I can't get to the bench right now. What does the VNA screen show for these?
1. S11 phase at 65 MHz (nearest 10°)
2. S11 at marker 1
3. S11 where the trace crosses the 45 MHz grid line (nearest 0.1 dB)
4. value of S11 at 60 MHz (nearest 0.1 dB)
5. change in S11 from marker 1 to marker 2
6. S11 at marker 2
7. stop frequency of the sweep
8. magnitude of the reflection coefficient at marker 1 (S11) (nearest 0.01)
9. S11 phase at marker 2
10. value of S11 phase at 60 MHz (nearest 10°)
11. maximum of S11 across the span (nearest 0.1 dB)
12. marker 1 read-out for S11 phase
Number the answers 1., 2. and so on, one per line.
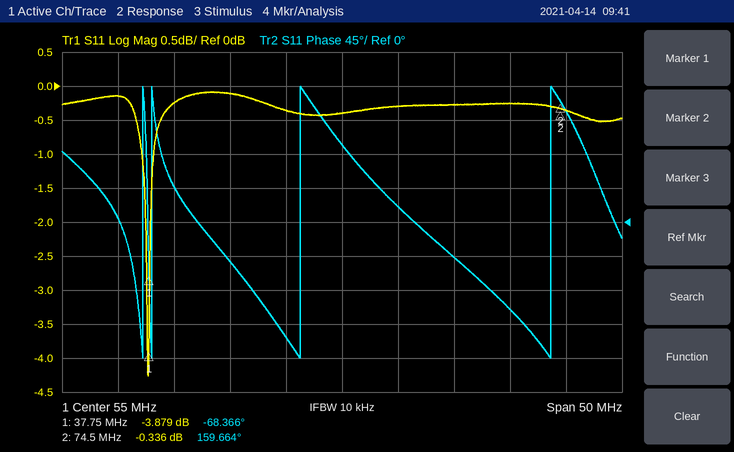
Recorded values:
1. -50°
2. -3.879 dB
3. -0.1 dB
4. -0.3 dB
5. 3.543 dB
6. -0.336 dB
7. 80 MHz
8. 0.64
9. 159.664°
10. 20°
11. -0.1 dB
12. -68.366°
